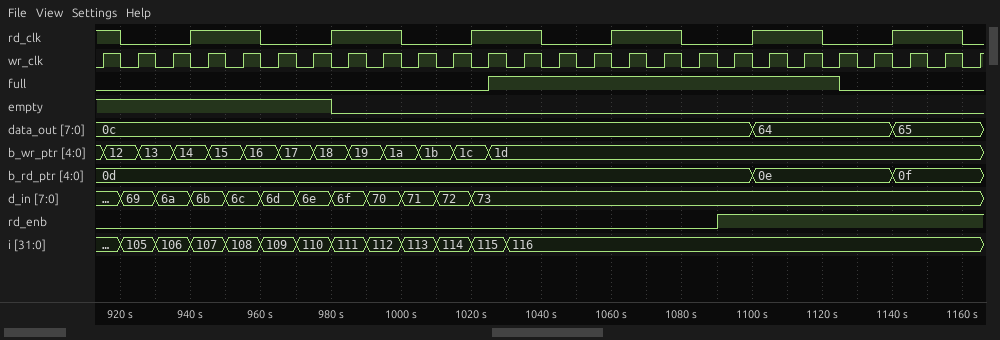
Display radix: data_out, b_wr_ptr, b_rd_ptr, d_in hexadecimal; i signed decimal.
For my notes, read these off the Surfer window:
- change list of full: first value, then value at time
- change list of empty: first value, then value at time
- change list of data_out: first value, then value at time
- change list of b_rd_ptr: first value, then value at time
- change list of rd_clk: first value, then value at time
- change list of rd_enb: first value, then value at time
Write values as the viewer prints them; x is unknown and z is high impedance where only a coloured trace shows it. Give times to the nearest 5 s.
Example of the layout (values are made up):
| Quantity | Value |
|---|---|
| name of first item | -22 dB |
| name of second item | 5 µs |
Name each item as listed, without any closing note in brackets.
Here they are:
| Quantity | Value |
|---|---|
| change list of full: first value, then value at time | 0, 1 at 1025 s, 0 at 1125 s |
| change list of empty: first value, then value at time | 1, 0 at 980 s |
| change list of data_out: first value, then value at time | 0c, 64 at 1100 s, 65 at 1140 s |
| change list of b_rd_ptr: first value, then value at time | 0d, 0e at 1100 s, 0f at 1140 s |
| change list of rd_clk: first value, then value at time | 1, 0 at 920 s, 1 at 940 s, 0 at 960 s, 1 at 980 s, 0 at 1000 s, 1 at 1020 s, 0 at 1040 s, 1 at 1060 s, 0 at 1080 s, 1 at 1100 s, 0 at 1120 s, 1 at 1140 s, 0 at 1160 s |
| change list of rd_enb: first value, then value at time | 0, 1 at 1090 s |
